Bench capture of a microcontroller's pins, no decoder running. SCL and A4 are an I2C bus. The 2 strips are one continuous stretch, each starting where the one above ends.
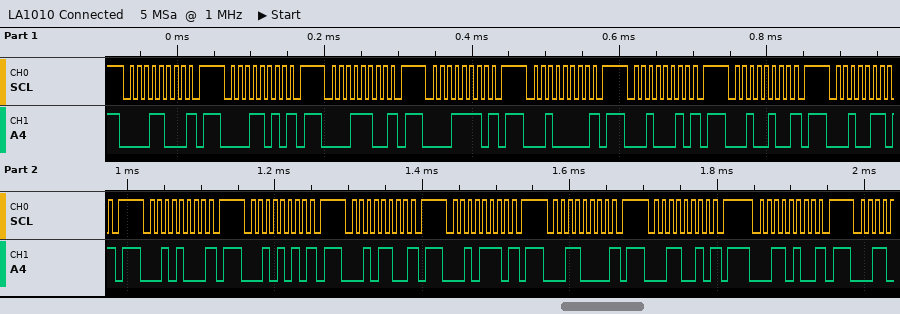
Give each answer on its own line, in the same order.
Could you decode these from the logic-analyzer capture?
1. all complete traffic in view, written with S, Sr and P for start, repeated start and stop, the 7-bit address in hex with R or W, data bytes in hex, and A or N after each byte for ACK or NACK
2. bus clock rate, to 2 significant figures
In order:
S 0CW N P S 0DW N P S 0EW N P S 0FW N P S 10W N P S 11W N P S 12W N P S 13W N P S 14W N P S 15W N P S 16W N P S 17W N P S 18W N P S 19W N P S 1AW N P
100 kHz
